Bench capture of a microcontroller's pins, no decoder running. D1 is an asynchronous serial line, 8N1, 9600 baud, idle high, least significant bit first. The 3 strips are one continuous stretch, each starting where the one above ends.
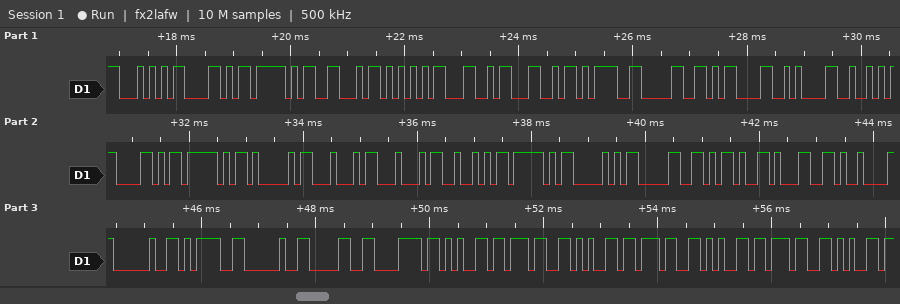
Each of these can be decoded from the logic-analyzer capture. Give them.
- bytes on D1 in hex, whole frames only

54 58 5F 46 55 4C 4C 3D 30 0D 0A 52 58 5F 41 44 44 52 5F 50 30 2D 31 09 20 3D 20 30 78 65 37 65 37 65 37 65
